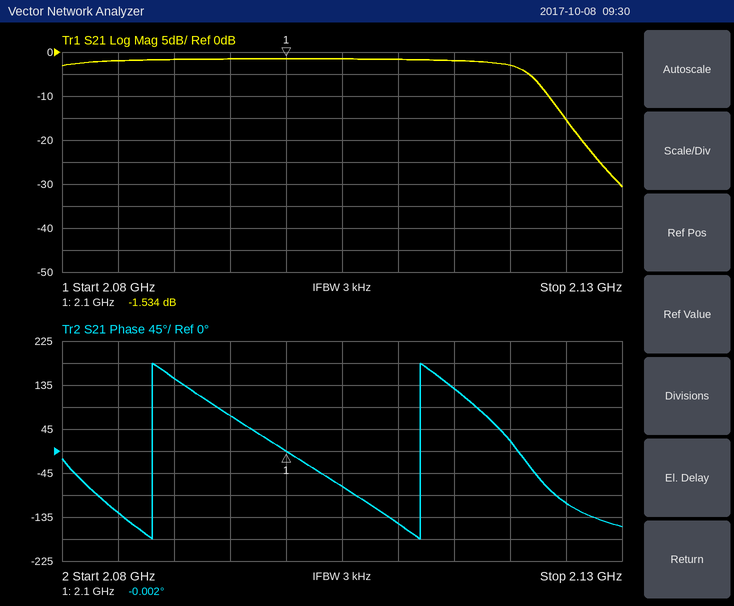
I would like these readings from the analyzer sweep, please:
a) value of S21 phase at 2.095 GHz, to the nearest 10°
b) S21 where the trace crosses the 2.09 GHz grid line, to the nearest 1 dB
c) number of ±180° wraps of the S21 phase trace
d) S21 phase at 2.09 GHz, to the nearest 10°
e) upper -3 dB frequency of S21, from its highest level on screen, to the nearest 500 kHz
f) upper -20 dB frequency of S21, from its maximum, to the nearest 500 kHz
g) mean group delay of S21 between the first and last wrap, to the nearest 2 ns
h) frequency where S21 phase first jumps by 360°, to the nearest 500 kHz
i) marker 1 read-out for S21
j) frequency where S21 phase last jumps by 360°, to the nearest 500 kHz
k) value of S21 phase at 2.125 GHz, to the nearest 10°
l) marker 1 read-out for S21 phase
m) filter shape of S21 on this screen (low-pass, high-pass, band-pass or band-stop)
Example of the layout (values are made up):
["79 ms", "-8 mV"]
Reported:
["70°", "-2 dB", "2", "150°", "2.1215 GHz", "2.1270 GHz", "42 ns", "2.0880 GHz", "-1.534 dB", "2.1120 GHz", "-110°", "-0.002°", "low-pass"]
